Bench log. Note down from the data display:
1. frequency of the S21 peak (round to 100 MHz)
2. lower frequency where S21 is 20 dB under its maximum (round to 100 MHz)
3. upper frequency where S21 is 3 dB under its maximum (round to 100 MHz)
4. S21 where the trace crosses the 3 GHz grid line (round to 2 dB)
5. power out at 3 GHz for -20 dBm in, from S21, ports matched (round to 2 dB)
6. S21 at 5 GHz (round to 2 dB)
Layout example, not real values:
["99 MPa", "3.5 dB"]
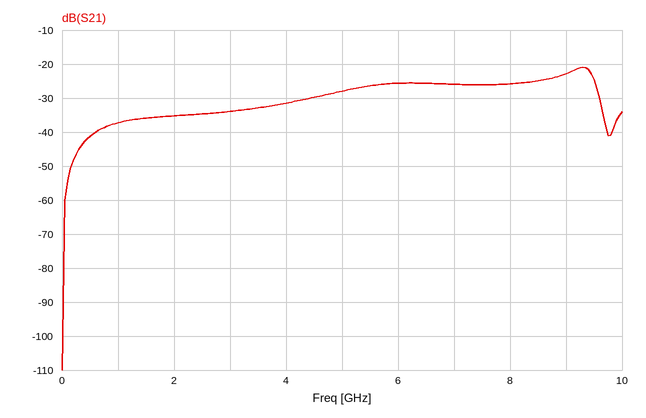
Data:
["9.3 GHz", "500 MHz", "9.5 GHz", "-34 dB", "-54 dBm", "-28 dB"]
